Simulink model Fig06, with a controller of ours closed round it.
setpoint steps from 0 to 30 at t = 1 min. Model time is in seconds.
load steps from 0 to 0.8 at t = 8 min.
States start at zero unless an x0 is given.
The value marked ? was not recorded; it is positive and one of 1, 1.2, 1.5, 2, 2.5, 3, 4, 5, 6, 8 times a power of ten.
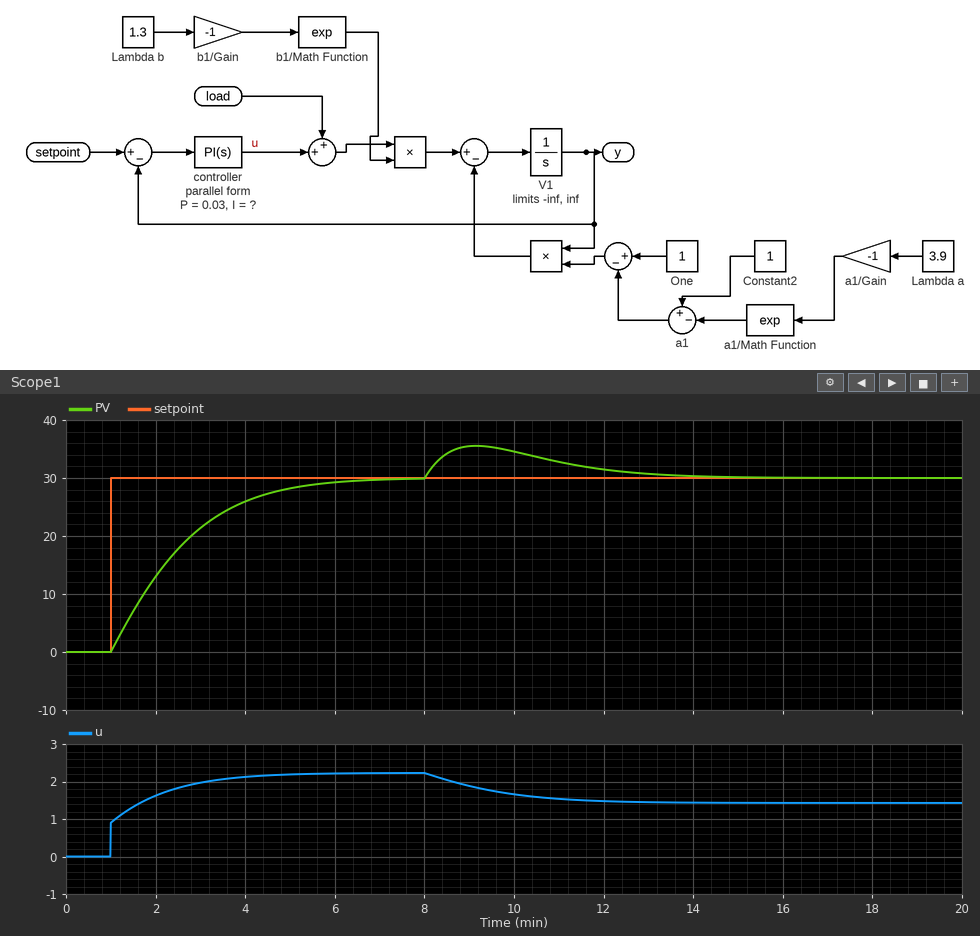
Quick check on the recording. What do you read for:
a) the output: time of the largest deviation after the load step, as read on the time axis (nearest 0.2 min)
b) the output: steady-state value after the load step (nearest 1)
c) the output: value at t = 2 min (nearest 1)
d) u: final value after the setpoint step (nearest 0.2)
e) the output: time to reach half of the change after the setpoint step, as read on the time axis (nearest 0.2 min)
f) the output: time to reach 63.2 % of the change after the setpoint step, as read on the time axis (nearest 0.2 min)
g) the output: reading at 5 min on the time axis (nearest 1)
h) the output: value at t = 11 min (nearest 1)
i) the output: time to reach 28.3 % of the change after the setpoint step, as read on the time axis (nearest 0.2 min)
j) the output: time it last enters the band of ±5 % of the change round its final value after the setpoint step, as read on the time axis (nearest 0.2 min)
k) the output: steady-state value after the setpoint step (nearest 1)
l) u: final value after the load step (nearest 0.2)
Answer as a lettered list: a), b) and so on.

a) 9.2 min
b) 30
c) 13
d) 2.2
e) 2.2 min
f) 2.6 min
g) 28
h) 33
i) 1.6 min
j) 5.2 min
k) 30
l) 1.4
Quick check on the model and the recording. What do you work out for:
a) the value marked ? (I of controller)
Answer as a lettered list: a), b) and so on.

a) 0.0008
